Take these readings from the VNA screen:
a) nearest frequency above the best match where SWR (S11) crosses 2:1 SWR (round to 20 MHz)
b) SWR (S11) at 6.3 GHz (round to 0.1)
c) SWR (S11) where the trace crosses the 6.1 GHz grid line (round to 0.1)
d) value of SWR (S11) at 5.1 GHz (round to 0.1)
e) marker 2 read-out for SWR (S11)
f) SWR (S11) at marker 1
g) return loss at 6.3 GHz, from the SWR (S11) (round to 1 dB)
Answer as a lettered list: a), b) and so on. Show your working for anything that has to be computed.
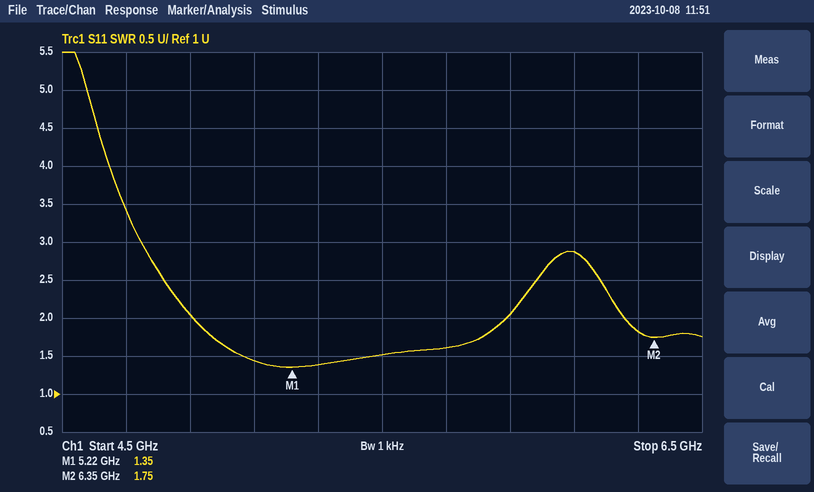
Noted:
a) 5.88 GHz
b) 1.8
c) 2.9
d) 1.4
e) 1.75
f) 1.35
g) −20 log10((1.8 − 1)/(1.8 + 1)) ≈ 11 dB
